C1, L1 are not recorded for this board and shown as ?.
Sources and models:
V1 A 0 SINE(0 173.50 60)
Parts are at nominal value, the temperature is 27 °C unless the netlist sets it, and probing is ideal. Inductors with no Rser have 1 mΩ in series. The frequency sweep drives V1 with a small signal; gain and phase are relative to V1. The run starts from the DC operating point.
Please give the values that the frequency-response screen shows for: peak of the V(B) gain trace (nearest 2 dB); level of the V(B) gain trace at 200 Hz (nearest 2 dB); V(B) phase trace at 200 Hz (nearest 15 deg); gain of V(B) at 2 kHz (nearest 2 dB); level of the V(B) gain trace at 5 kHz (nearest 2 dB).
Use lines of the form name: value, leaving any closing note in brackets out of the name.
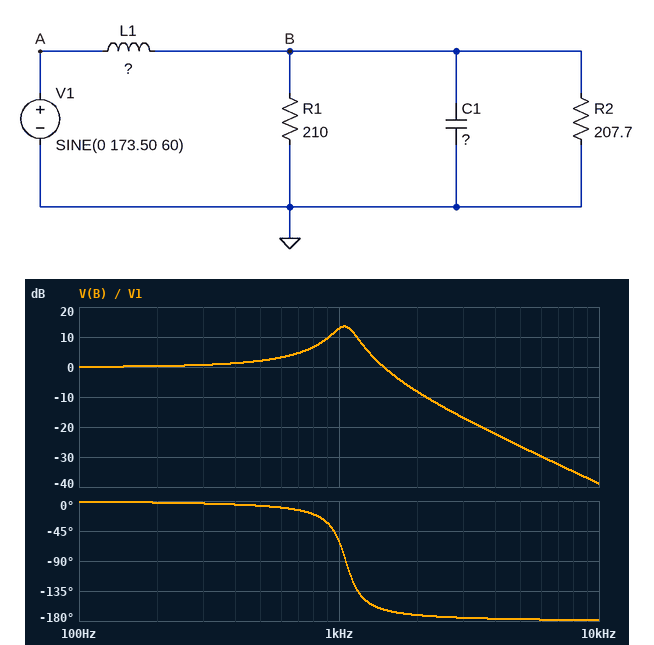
peak of the V(B) gain trace: 14 dB
level of the V(B) gain trace at 200 Hz: 0 dB
V(B) phase trace at 200 Hz: 0 deg
gain of V(B) at 2 kHz: -8 dB
level of the V(B) gain trace at 5 kHz: -26 dB
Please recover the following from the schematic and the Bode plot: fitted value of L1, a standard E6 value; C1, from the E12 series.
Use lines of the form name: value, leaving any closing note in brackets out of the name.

fitted value of L1, a standard E6 value: 3.3 mH
C1, from the E12 series: 6.8 µF
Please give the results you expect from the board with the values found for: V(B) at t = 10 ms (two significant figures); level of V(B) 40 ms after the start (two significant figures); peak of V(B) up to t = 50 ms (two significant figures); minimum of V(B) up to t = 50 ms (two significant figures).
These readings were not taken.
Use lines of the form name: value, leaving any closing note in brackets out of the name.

V(B) at t = 10 ms: -100 V
level of V(B) 40 ms after the start: 100 V
peak of V(B) up to t = 50 ms: 170 V
minimum of V(B) up to t = 50 ms: -170 V
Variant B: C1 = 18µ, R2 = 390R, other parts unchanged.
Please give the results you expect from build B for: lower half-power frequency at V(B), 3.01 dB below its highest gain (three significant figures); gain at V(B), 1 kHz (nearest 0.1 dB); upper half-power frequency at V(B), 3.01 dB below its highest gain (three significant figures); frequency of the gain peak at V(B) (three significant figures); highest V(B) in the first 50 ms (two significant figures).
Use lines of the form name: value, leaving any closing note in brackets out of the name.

lower half-power frequency at V(B), 3.01 dB below its highest gain: 618 Hz
gain at V(B), 1 kHz: -2.6 dB
upper half-power frequency at V(B), 3.01 dB below its highest gain: 683 Hz
frequency of the gain peak at V(B): 651 Hz
highest V(B) in the first 50 ms: 180 V
